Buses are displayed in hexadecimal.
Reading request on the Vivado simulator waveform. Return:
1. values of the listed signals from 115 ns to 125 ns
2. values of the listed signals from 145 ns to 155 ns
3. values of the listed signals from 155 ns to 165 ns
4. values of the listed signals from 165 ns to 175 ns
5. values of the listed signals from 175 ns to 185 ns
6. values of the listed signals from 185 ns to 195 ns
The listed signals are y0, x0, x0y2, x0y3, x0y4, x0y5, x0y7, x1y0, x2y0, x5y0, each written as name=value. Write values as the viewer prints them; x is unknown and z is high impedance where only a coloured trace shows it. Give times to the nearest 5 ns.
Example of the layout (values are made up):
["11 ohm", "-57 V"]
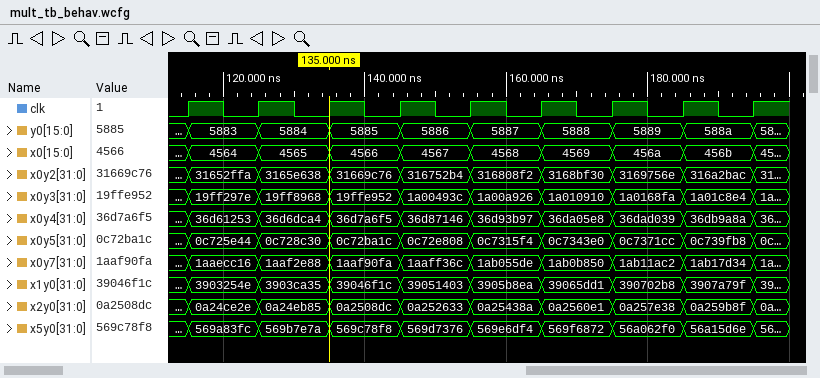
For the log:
["y0=5883, x0=4564, x0y2=31652ffa, x0y3=19ff297e, x0y4=36d61253, x0y5=0c725e44, x0y7=1aaecc16, x1y0=3903254e, x2y0=0a24ce2e, x5y0=569a83fc", "y0=5886, x0=4567, x0y2=316752b4, x0y3=1a00493c, x0y4=36d87146, x0y5=0c72e808, x0y7=1aaff36c, x1y0=39051403, x2y0=0a252633, x5y0=569d7376", "y0=5887, x0=4568, x0y2=316808f2, x0y3=1a00a926, x0y4=36d93b97, x0y5=0c7315f4, x0y7=1ab055de, x1y0=3905b8ea, x2y0=0a25438a, x5y0=569e6df4", "y0=5888, x0=4569, x0y2=3168bf30, x0y3=1a010910, x0y4=36da05e8, x0y5=0c7343e0, x0y7=1ab0b850, x1y0=39065dd1, x2y0=0a2560e1, x5y0=569f6872", "y0=5889, x0=456a, x0y2=3169756e, x0y3=1a0168fa, x0y4=36dad039, x0y5=0c7371cc, x0y7=1ab11ac2, x1y0=390702b8, x2y0=0a257e38, x5y0=56a062f0", "y0=588a, x0=456b, x0y2=316a2bac, x0y3=1a01c8e4, x0y4=36db9a8a, x0y5=0c739fb8, x0y7=1ab17d34, x1y0=3907a79f, x2y0=0a259b8f, x5y0=56a15d6e"]
